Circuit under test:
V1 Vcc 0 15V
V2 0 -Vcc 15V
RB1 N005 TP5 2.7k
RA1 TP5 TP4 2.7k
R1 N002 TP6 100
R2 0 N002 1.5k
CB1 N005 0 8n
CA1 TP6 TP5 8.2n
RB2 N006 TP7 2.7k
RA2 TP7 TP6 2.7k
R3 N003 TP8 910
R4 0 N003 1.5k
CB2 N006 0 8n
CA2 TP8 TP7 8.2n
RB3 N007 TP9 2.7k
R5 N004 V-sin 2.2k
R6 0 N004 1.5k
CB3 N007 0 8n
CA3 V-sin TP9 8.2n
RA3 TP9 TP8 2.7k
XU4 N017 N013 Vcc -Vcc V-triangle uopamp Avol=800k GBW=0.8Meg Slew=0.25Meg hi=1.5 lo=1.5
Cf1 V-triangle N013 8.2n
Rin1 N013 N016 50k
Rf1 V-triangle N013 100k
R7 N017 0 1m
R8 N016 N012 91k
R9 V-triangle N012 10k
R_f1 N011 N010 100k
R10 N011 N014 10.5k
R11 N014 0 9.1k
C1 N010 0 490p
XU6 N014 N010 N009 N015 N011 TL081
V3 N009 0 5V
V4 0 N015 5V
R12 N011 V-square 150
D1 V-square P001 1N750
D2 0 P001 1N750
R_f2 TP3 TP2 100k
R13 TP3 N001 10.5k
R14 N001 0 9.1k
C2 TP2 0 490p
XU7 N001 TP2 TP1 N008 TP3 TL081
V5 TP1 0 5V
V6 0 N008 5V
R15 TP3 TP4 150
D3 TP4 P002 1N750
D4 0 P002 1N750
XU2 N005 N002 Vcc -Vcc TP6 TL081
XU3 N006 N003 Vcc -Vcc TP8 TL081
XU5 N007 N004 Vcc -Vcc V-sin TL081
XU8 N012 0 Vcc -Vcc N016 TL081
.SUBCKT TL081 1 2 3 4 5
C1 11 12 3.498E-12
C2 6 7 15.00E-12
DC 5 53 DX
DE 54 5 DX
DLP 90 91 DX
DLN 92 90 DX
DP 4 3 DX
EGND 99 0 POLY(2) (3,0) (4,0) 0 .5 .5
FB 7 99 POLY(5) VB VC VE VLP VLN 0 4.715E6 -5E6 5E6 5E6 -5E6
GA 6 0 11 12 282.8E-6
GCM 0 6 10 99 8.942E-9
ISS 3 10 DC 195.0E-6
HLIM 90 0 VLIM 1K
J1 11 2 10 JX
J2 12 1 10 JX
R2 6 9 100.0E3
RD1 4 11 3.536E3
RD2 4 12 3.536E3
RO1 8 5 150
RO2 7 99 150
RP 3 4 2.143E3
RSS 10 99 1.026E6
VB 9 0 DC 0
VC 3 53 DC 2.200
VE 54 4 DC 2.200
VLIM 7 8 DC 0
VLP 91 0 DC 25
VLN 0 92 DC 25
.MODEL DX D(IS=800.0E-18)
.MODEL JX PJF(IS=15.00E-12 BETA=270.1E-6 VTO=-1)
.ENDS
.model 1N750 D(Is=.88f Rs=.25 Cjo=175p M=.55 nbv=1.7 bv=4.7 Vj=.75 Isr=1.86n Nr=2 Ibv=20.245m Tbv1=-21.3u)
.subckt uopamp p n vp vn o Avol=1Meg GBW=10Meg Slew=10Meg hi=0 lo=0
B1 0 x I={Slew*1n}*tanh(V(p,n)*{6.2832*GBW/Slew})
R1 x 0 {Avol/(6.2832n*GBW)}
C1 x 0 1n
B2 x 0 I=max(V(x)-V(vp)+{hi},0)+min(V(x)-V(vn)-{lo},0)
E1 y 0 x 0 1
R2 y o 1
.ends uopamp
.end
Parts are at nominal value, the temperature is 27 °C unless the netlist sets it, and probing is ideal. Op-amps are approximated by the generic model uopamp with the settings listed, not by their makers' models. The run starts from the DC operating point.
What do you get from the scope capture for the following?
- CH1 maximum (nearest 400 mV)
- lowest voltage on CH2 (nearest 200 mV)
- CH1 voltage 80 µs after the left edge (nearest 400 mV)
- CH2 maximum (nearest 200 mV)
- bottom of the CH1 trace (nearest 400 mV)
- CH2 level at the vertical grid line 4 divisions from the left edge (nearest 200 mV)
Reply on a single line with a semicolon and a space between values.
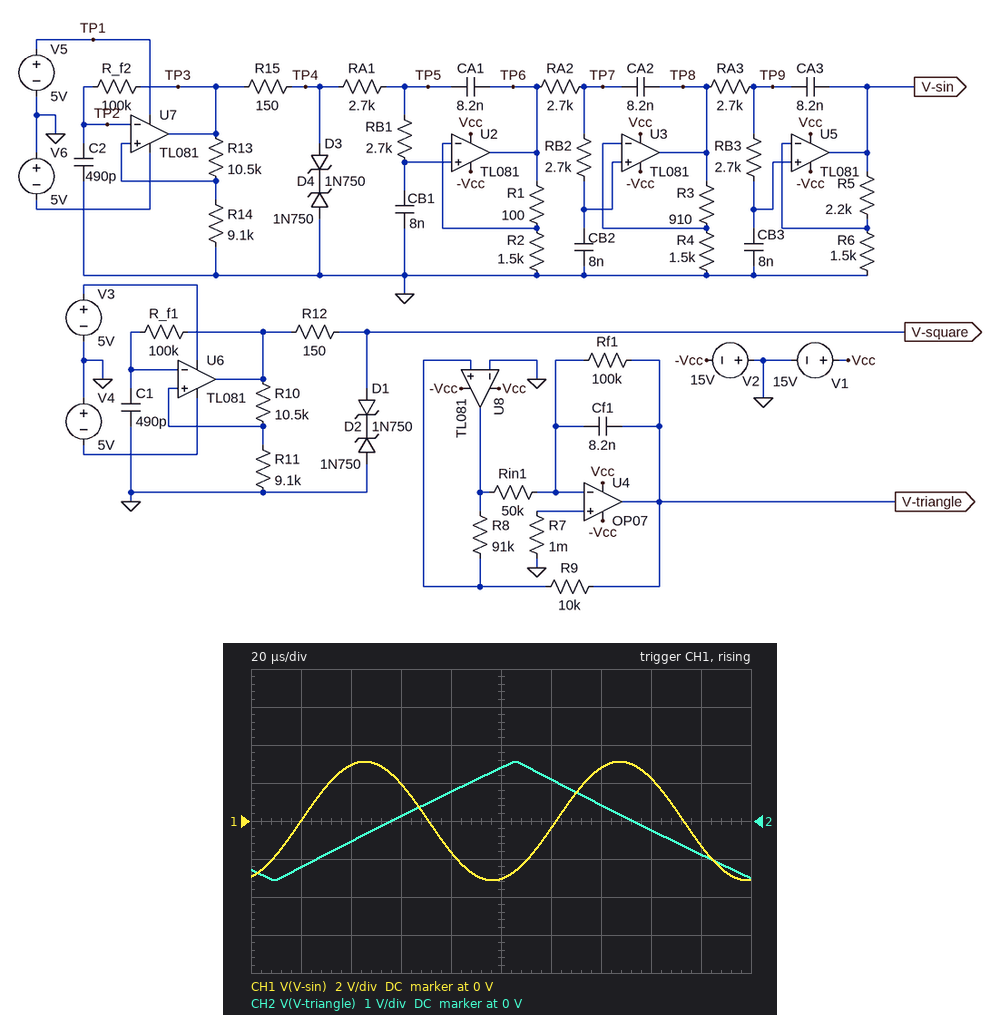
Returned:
3.2 V; -1.6 V; -1.6 V; 1.6 V; -3.2 V; 800 mV
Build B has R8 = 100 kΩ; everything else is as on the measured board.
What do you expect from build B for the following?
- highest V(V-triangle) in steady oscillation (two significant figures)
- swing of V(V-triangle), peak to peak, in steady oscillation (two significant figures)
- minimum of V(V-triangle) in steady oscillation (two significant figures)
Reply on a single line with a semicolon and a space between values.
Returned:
1.4 V; 2.9 V; -1.4 V
